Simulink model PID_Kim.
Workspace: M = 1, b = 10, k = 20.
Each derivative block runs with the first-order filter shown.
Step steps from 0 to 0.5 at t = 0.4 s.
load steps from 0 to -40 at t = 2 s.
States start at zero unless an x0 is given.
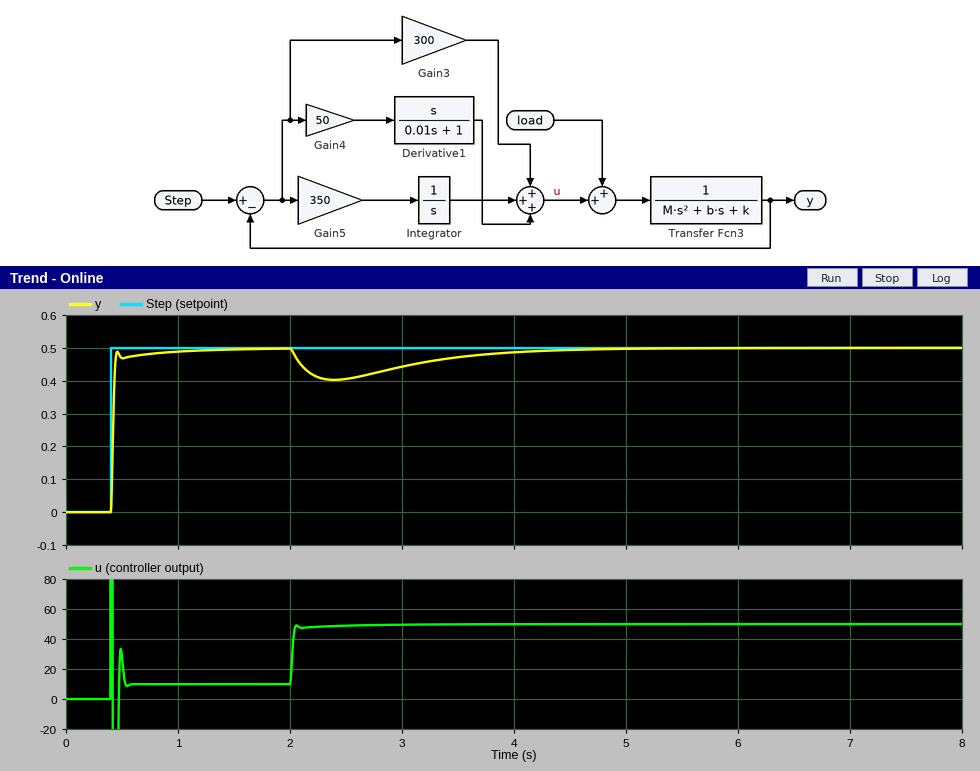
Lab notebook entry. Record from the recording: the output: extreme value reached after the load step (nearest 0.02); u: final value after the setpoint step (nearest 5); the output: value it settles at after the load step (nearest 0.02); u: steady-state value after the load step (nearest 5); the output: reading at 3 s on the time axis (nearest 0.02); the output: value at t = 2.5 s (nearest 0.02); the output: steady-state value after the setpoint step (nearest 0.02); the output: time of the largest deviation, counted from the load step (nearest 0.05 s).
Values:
0.40
10
0.50
50
0.44
0.40
0.50
0.40 s
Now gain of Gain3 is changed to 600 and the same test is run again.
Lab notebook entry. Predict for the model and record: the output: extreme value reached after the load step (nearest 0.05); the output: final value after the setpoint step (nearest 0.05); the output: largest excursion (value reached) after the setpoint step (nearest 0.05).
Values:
0.45
0.50
0.55
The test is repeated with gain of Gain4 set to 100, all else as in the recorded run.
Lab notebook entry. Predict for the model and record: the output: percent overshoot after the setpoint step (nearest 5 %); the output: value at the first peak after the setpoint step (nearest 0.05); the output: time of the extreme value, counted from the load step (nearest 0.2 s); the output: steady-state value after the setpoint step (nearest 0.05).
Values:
10 %
0.55
0.6 s
0.50
